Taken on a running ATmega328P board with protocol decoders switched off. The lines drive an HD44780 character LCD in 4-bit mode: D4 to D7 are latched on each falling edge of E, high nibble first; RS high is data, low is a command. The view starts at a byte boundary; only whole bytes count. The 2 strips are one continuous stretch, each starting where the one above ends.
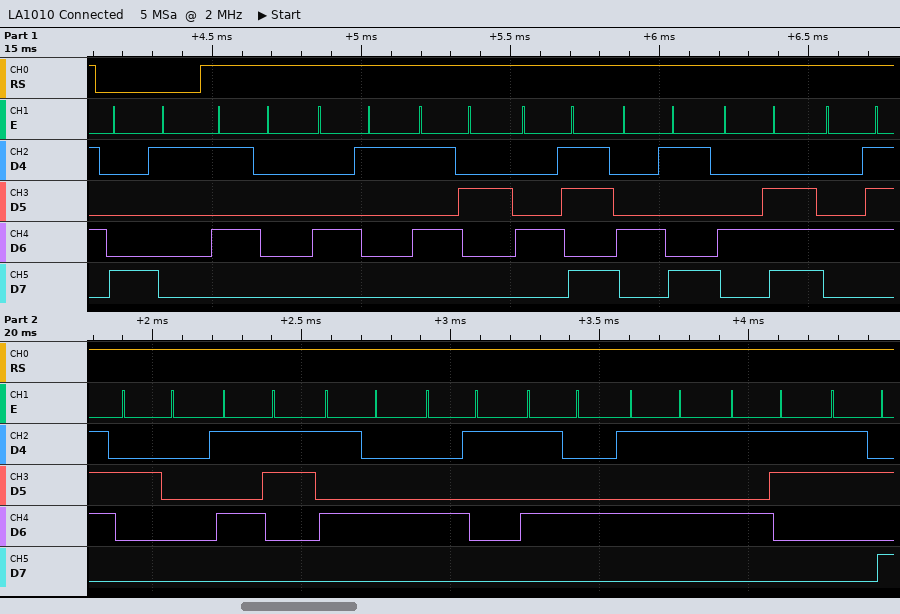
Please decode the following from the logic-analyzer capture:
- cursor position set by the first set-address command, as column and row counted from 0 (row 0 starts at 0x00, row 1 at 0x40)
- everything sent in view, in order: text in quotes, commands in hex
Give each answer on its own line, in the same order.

column 1, row 0
0x81 "PARKING STATUS:"
